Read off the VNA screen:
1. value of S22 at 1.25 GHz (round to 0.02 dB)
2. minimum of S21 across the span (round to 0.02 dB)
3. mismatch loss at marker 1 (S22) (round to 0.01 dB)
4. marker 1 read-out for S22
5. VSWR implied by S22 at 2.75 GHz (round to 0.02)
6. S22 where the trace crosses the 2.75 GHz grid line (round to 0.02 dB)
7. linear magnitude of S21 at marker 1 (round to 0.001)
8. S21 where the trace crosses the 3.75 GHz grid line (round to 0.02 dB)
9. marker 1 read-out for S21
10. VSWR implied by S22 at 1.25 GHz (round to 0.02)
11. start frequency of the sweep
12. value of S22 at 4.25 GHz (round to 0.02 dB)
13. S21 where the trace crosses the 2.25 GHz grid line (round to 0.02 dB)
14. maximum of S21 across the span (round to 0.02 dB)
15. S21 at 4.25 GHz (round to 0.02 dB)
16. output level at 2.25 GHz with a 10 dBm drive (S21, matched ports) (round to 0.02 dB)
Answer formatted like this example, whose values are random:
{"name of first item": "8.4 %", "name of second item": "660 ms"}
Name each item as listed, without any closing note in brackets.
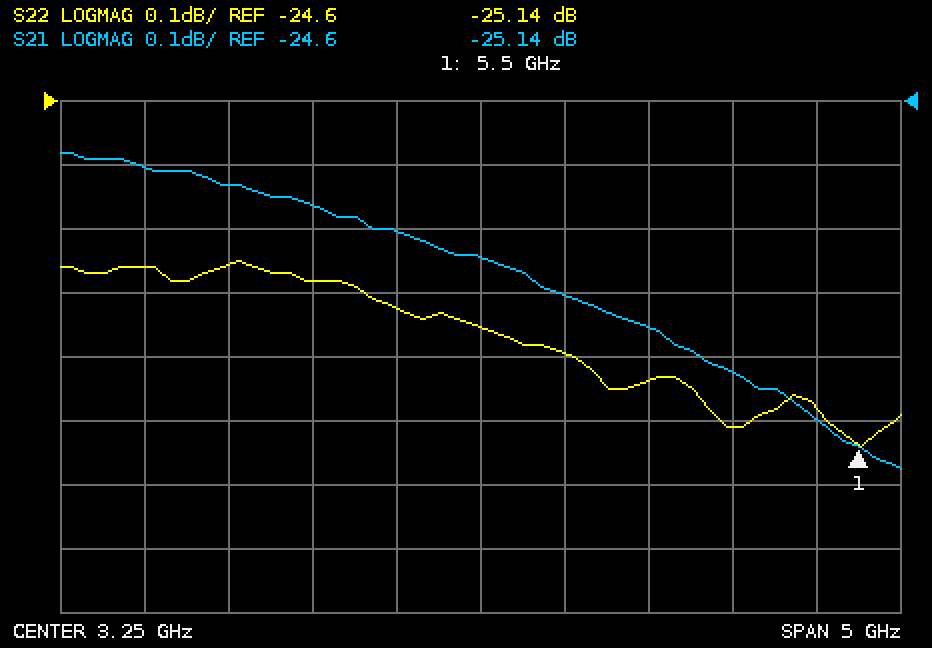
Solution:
{"value of S22 at 1.25 GHz": "-24.86 dB", "minimum of S21 across the span": "-25.18 dB", "mismatch loss at marker 1 (S22)": "0.01 dB", "marker 1 read-out for S22": "-25.14 dB", "VSWR implied by S22 at 2.75 GHz": "1.12", "S22 where the trace crosses the 2.75 GHz grid line": "-24.92 dB", "linear magnitude of S21 at marker 1": "0.055", "S21 where the trace crosses the 3.75 GHz grid line": "-24.90 dB", "marker 1 read-out for S21": "-25.14 dB", "VSWR implied by S22 at 1.25 GHz": "1.12", "start frequency of the sweep": "750 MHz", "value of S22 at 4.25 GHz": "-25.04 dB", "S21 where the trace crosses the 2.25 GHz grid line": "-24.76 dB", "maximum of S21 across the span": "-24.68 dB", "S21 at 4.25 GHz": "-24.96 dB", "output level at 2.25 GHz with a 10 dBm drive (S21, matched ports)": "-14.76 dBm"}
